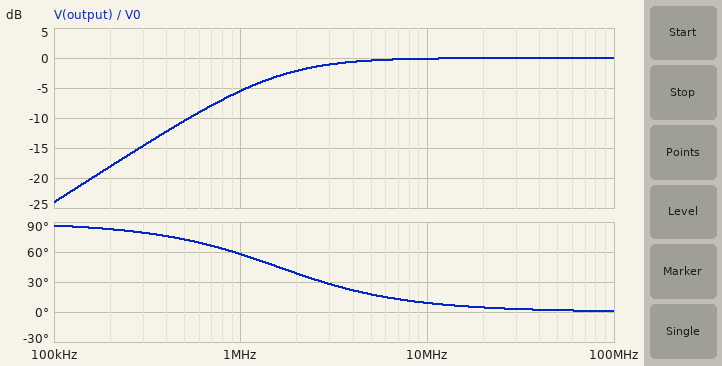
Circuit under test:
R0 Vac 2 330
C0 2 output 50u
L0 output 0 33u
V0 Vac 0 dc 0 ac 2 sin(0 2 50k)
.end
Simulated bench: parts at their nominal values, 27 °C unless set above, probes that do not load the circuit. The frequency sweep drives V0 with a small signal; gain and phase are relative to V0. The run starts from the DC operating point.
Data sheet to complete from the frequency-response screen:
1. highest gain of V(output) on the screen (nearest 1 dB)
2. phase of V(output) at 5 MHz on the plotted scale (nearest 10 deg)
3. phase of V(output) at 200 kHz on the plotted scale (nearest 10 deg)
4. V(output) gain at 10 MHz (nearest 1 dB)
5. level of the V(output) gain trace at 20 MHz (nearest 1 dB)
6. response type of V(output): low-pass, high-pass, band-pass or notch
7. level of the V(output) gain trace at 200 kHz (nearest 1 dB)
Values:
0 dB
20 deg
80 deg
0 dB
0 dB
high-pass
-18 dB
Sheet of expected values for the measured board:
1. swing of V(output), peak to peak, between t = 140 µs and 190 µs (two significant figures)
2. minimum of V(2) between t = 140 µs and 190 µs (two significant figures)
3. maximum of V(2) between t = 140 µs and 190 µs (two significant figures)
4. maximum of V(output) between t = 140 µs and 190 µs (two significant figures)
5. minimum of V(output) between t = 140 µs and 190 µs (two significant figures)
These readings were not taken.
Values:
130 mV
-62 mV
63 mV
63 mV
-63 mV
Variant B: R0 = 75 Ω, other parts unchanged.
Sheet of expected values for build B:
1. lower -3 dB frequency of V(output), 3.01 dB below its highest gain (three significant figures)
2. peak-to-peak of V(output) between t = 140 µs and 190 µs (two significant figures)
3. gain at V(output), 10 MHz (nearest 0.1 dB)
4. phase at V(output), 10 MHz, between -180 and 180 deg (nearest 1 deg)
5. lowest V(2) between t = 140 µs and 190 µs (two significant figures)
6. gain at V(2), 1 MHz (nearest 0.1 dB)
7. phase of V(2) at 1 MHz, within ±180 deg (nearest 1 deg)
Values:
362 kHz
550 mV
0 dB
2 deg
-270 mV
-0.5 dB
20 deg
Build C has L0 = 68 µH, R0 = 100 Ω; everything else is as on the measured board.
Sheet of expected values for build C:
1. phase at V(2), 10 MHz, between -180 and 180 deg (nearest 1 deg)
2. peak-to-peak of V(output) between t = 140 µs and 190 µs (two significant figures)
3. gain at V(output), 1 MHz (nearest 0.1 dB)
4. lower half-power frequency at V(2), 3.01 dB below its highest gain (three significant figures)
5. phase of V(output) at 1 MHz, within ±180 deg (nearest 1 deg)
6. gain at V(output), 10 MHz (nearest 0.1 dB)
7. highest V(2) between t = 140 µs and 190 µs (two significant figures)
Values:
1 deg
840 mV
-0.2 dB
234 kHz
13 deg
0 dB
420 mV
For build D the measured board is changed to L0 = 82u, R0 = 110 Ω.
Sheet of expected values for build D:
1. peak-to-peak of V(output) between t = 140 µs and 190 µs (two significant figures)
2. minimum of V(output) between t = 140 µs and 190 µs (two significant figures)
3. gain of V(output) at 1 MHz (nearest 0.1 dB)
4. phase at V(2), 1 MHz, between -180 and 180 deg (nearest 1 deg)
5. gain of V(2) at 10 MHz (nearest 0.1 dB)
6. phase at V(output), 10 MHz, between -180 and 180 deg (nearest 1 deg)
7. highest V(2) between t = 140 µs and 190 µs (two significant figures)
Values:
910 mV
-460 mV
-0.2 dB
12 deg
0 dB
1 deg
460 mV
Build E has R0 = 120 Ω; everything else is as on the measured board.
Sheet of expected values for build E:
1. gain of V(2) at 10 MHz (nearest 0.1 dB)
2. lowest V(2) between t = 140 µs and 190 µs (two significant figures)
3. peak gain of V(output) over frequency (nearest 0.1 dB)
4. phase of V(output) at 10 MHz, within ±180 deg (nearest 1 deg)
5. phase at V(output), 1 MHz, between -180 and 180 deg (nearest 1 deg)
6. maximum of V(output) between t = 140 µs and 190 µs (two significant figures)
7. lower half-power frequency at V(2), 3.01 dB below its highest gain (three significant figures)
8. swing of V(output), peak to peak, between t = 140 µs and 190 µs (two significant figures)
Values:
0 dB
-170 mV
0 dB
3 deg
30 deg
170 mV
579 kHz
340 mV
